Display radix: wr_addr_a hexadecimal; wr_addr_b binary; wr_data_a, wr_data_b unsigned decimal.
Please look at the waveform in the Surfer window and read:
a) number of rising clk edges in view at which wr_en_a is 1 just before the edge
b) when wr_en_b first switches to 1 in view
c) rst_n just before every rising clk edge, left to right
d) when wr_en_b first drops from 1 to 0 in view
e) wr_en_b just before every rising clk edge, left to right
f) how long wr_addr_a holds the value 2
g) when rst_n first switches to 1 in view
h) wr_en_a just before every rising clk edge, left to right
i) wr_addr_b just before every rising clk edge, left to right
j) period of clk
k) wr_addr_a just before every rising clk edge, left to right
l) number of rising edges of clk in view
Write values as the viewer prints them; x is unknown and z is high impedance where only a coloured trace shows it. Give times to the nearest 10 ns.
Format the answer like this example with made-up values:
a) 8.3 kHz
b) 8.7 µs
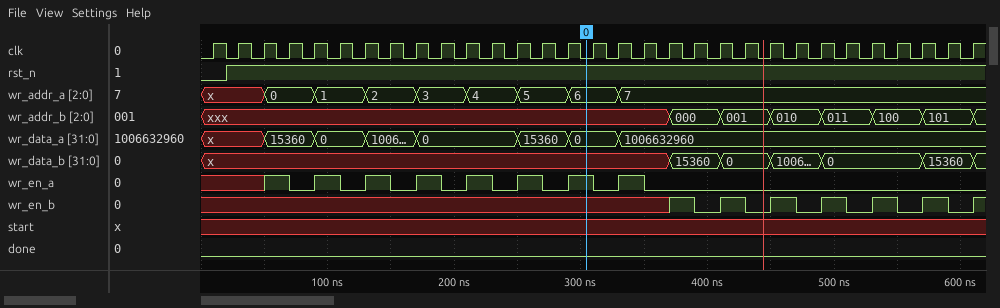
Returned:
a) 8
b) 370 ns
c) 0 1 1 1 1 1 1 1 1 1 1 1 1 1 1 1 1 1 1 1 1 1 1 1 1 1 1 1 1 1 1
d) 390 ns
e) x x x x x x x x x x x x x x x x x x x 1 0 1 0 1 0 1 0 1 0 1 0
f) 40 ns
g) 20 ns
h) x x x 1 0 1 0 1 0 1 0 1 0 1 0 1 0 1 0 0 0 0 0 0 0 0 0 0 0 0 0
i) xxx, xxx, xxx, xxx, xxx, xxx, xxx, xxx, xxx, xxx, xxx, xxx, xxx, xxx, xxx, xxx, xxx, xxx, xxx, 000, 000, 001, 001, 010, 010, 011, 011, 100, 100, 101, 101
j) 20 ns
k) x, x, x, 0, 0, 1, 1, 2, 2, 3, 3, 4, 4, 5, 5, 6, 6, 7, 7, 7, 7, 7, 7, 7, 7, 7, 7, 7, 7, 7, 7
l) 31
